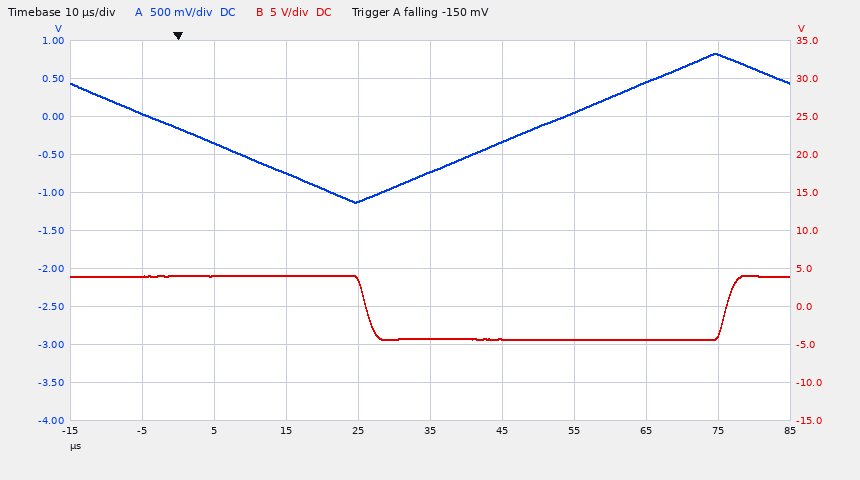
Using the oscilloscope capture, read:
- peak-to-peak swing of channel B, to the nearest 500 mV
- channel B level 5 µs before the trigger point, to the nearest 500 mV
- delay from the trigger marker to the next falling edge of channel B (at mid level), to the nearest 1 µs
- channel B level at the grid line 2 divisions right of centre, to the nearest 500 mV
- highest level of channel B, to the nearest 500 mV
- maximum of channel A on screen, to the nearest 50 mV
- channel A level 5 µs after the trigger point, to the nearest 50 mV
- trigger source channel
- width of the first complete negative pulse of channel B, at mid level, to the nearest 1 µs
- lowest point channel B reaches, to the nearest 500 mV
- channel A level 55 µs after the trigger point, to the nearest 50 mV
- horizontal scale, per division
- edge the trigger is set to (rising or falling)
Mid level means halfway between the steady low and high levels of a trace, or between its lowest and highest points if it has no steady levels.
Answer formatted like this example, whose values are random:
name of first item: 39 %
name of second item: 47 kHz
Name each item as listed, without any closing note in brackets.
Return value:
peak-to-peak swing of channel B, to the nearest 500 mV: 8.5 V
channel B level 5 µs before the trigger point, to the nearest 500 mV: 4.0 V
delay from the trigger marker to the next falling edge of channel B (at mid level), to the nearest 1 µs: 26 µs
channel B level at the grid line 2 divisions right of centre, to the nearest 500 mV: -4.5 V
highest level of channel B, to the nearest 500 mV: 4.0 V
maximum of channel A on screen, to the nearest 50 mV: 850 mV
channel A level 5 µs after the trigger point, to the nearest 50 mV: -350 mV
trigger source channel: channel A
width of the first complete negative pulse of channel B, at mid level, to the nearest 1 µs: 50 µs
lowest point channel B reaches, to the nearest 500 mV: -4.5 V
channel A level 55 µs after the trigger point, to the nearest 50 mV: 50 mV
horizontal scale, per division: 10 µs
edge the trigger is set to: falling
